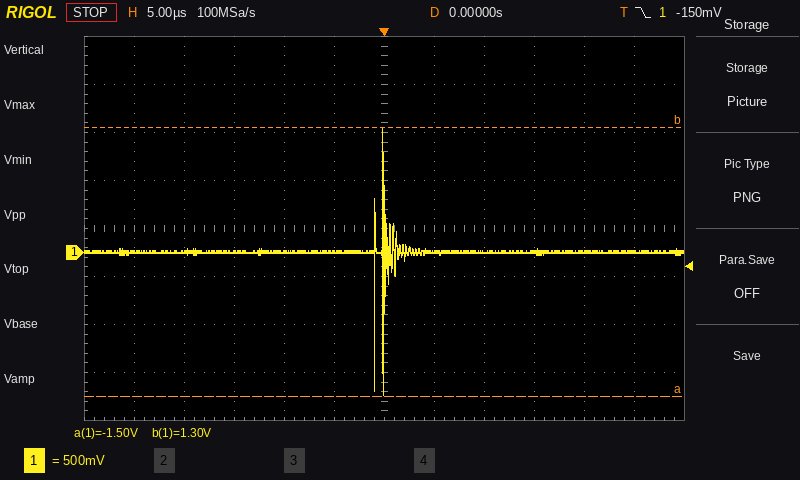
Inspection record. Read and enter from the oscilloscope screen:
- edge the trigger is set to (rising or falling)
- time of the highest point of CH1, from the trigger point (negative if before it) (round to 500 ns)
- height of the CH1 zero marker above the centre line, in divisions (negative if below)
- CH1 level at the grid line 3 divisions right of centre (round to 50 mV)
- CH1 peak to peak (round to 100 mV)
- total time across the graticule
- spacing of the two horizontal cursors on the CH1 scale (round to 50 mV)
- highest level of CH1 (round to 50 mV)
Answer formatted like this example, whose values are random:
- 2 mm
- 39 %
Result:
- falling
- 0.0 µs
- -0.5 div
- 0 mV
- 2.80 V
- 60 µs
- 2.80 V
- 1.30 V
